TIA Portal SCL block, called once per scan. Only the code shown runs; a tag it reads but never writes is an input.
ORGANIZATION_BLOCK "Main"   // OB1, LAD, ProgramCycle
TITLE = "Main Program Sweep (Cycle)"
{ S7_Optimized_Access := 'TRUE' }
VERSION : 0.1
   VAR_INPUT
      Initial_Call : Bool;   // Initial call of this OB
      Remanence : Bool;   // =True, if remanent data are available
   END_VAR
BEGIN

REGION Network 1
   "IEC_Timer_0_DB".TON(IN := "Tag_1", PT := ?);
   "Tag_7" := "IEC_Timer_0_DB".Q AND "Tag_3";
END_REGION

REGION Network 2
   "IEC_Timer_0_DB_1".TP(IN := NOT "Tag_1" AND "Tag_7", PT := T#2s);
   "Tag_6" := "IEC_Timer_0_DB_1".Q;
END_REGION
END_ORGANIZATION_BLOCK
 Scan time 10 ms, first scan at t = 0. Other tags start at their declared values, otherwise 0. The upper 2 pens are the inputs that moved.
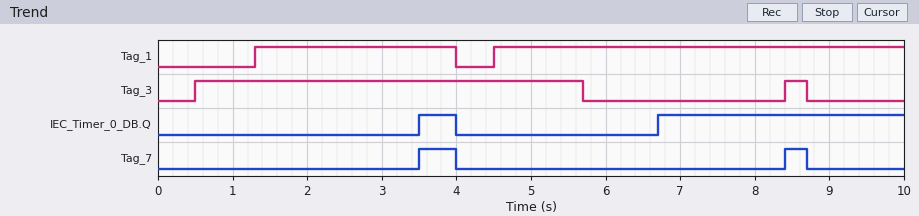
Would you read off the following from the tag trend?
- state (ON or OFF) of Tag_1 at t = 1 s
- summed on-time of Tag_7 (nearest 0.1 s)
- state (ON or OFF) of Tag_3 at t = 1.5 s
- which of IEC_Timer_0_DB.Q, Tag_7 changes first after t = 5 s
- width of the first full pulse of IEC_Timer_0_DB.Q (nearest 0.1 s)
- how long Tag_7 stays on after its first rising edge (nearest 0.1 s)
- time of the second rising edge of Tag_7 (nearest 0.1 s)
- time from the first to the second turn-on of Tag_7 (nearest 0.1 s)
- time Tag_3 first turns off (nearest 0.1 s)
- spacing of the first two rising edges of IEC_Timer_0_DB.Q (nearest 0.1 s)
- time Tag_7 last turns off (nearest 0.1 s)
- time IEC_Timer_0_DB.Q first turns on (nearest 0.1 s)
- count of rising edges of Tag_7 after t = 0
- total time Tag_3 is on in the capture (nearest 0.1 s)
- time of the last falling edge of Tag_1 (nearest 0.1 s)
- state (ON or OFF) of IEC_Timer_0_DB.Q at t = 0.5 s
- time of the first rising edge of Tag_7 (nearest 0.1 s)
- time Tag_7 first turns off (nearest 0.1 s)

OFF
0.8 s
ON
IEC_Timer_0_DB.Q
0.5 s
0.5 s
8.4 s
4.9 s
5.7 s
3.2 s
8.7 s
3.5 s
2
5.5 s
4.0 s
OFF
3.5 s
4.0 s
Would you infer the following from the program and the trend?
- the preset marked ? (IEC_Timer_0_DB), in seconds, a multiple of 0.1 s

2.2 s
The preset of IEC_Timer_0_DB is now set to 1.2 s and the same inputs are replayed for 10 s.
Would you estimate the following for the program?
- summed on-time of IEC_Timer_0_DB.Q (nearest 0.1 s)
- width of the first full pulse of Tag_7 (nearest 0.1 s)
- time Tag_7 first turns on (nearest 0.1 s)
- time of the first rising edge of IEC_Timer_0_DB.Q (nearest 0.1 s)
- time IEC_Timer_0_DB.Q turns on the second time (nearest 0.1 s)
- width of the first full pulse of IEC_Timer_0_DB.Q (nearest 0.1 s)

5.8 s
1.5 s
2.5 s
2.5 s
5.7 s
1.5 s
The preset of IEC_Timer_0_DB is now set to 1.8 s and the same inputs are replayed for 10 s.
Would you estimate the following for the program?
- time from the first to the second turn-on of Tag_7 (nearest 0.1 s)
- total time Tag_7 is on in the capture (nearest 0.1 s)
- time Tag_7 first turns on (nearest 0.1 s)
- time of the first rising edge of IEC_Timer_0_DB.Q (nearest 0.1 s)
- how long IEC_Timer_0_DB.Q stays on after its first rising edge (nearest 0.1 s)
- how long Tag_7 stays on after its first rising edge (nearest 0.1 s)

5.3 s
1.2 s
3.1 s
3.1 s
0.9 s
0.9 s
